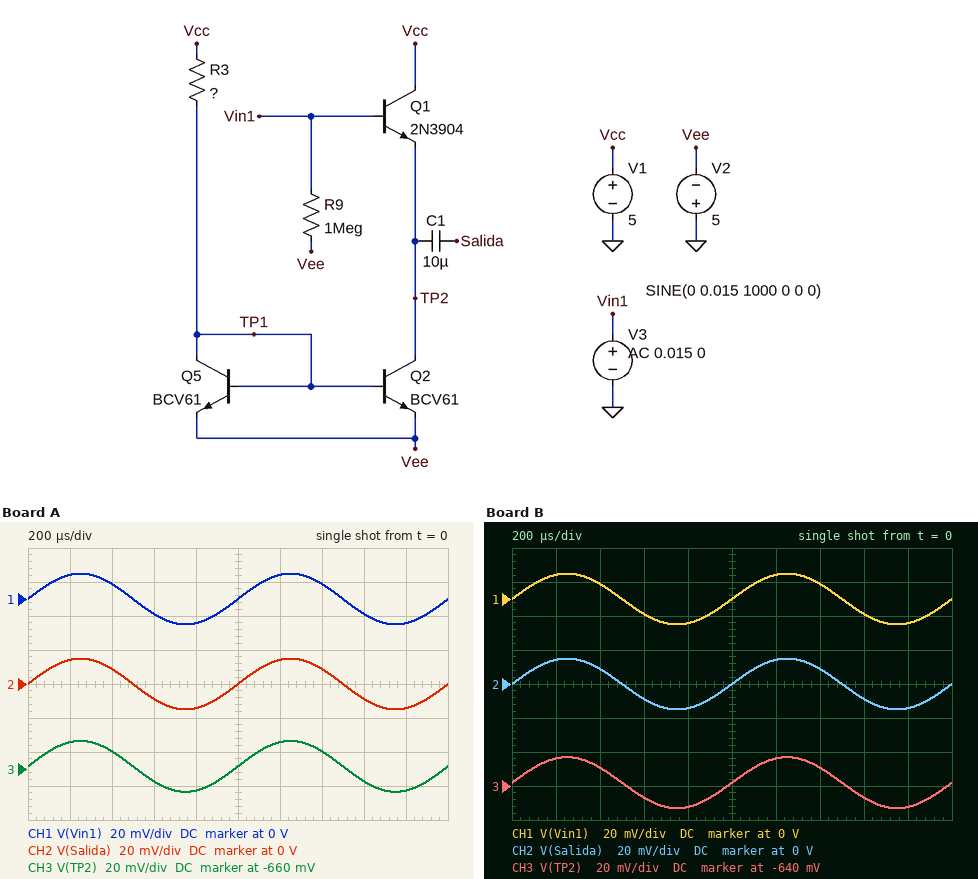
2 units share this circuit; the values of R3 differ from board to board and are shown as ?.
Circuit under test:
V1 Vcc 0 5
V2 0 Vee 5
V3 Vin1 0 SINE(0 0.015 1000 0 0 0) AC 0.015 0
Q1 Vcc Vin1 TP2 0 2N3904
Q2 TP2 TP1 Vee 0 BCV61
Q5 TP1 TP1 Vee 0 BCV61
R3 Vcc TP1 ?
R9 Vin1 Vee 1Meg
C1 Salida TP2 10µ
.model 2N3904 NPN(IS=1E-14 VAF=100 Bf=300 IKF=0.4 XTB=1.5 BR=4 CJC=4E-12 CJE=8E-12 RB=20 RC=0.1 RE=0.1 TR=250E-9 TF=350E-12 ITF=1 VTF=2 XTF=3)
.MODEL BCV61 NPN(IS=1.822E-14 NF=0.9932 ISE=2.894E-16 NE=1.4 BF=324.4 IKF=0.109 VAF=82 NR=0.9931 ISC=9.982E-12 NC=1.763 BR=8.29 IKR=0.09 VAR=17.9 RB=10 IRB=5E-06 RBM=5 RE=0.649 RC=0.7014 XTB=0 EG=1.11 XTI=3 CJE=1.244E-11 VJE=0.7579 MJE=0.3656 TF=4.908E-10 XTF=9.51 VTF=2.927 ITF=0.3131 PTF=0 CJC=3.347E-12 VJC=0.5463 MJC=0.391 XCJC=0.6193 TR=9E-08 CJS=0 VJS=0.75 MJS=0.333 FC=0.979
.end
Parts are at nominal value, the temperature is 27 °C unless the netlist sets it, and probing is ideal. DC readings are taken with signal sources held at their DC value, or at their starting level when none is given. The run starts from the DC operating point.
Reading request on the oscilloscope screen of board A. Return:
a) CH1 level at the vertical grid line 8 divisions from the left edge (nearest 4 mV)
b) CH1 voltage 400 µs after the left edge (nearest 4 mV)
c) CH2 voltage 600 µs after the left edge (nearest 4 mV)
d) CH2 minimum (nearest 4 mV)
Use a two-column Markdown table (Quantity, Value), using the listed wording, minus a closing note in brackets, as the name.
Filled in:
| Quantity | Value |
|---|---|
| CH1 level at the vertical grid line 8 divisions from the left edge | -8 mV |
| CH1 voltage 400 µs after the left edge | 8 mV |
| CH2 voltage 600 µs after the left edge | -8 mV |
| CH2 minimum | -16 mV |
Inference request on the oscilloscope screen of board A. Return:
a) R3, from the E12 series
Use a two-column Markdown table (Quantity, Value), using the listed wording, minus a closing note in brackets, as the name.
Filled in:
| Quantity | Value |
|---|---|
| R3, from the E12 series | 8.2 kΩ |
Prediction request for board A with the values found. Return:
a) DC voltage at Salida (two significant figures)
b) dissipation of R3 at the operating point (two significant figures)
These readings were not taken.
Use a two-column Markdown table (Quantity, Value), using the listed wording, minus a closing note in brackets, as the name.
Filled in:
| Quantity | Value |
|---|---|
| DC voltage at Salida | -660 mV |
| dissipation of R3 at the operating point | 11 mW |
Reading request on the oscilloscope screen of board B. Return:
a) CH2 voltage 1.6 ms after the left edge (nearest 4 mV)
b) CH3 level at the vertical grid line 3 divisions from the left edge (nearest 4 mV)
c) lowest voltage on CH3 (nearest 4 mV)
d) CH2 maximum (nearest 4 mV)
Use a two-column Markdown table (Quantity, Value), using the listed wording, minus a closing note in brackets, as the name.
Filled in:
| Quantity | Value |
|---|---|
| CH2 voltage 1.6 ms after the left edge | -8 mV |
| CH3 level at the vertical grid line 3 divisions from the left edge | -648 mV |
| lowest voltage on CH3 | -652 mV |
| CH2 maximum | 16 mV |
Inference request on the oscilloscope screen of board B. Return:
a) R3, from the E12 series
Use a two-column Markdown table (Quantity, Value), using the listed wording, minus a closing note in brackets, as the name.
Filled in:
| Quantity | Value |
|---|---|
| R3, from the E12 series | 18 kΩ |
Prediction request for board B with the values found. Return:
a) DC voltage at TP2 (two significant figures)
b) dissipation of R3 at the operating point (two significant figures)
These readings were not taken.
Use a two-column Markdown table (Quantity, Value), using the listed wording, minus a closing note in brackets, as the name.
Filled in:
| Quantity | Value |
|---|---|
| DC voltage at TP2 | -640 mV |
| dissipation of R3 at the operating point | 4.9 mW |
